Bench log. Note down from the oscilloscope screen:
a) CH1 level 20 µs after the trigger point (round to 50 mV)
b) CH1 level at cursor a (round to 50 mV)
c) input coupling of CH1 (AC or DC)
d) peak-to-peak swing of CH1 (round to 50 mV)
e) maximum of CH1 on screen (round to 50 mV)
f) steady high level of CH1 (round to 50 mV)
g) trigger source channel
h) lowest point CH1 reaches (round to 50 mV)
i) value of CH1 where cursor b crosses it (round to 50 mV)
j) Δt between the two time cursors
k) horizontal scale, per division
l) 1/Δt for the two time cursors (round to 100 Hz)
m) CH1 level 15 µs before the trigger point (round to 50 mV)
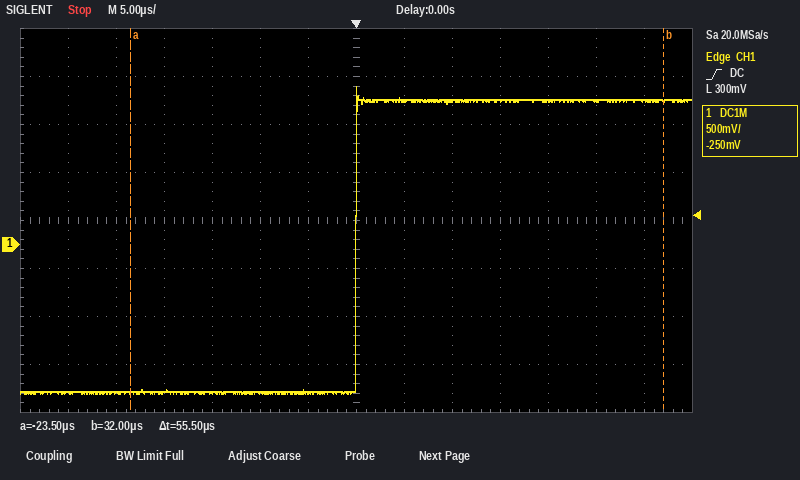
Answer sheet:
1.50 V
-1.55 V
DC
3.20 V
1.65 V
1.50 V
CH1
-1.55 V
1.50 V
55.5 µs
5 µs
18.0 kHz
-1.55 V
